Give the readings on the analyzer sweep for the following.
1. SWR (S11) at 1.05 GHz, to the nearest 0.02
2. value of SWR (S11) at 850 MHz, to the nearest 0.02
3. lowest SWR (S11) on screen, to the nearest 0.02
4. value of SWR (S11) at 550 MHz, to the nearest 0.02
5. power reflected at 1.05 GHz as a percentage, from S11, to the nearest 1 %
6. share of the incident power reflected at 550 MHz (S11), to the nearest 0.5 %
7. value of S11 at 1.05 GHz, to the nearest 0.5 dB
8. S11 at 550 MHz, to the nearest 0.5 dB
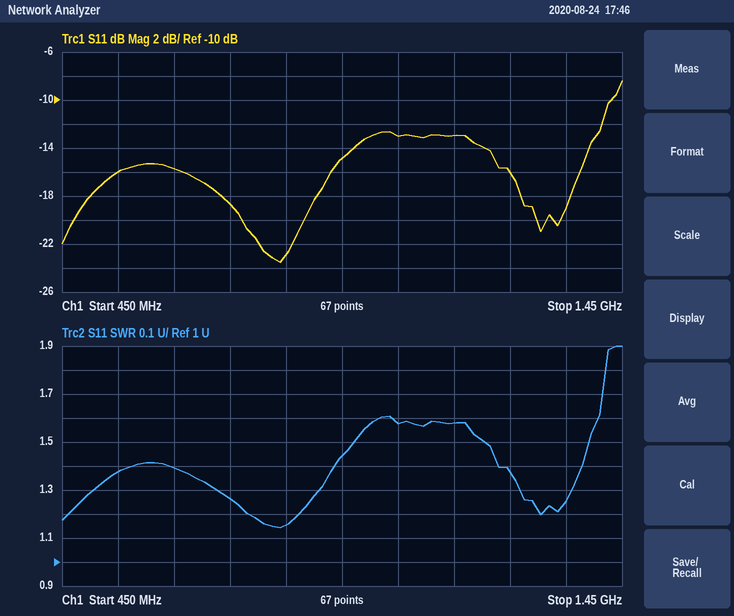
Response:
1.58
1.16
1.14
1.38
5 %
2.5 %
-13.0 dB
-16.0 dB
